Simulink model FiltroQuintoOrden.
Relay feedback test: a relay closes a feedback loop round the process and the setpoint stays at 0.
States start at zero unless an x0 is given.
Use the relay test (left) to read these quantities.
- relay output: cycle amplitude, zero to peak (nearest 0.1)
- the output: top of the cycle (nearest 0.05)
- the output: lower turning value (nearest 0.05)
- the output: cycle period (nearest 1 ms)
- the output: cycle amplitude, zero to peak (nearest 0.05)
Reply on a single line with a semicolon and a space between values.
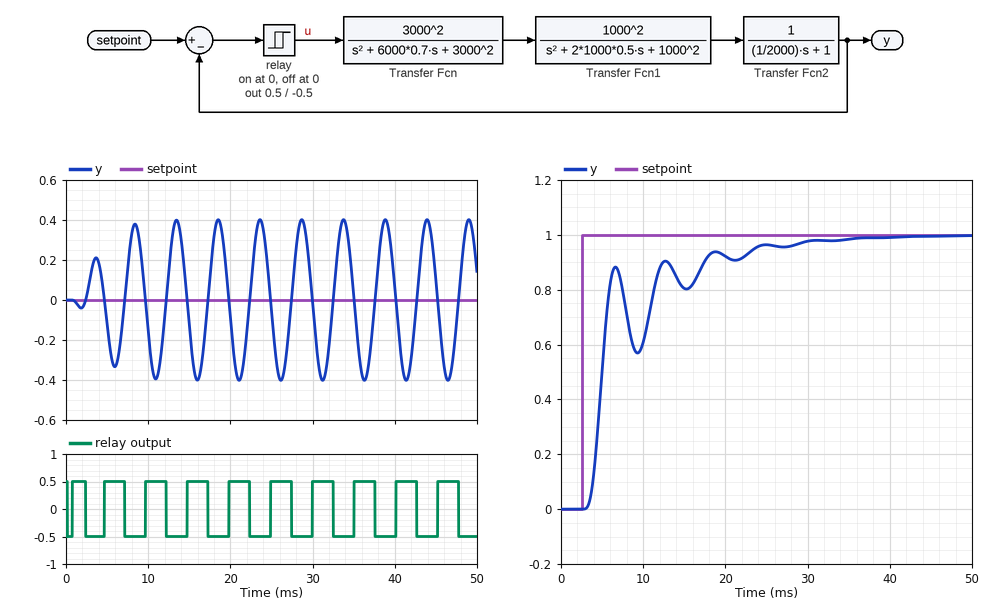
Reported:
0.5; 0.40; -0.40; 5 ms; 0.40
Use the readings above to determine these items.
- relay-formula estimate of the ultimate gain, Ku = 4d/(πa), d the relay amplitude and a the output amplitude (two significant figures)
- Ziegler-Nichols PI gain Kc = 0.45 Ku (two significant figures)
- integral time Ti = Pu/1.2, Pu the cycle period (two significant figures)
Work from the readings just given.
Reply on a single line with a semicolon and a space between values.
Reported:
1.6; 0.72; 4.2 ms
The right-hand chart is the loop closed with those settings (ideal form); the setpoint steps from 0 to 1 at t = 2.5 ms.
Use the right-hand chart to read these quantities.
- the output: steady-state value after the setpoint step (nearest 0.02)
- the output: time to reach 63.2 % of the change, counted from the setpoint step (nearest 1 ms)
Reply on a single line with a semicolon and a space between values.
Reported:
1.00; 3 ms
